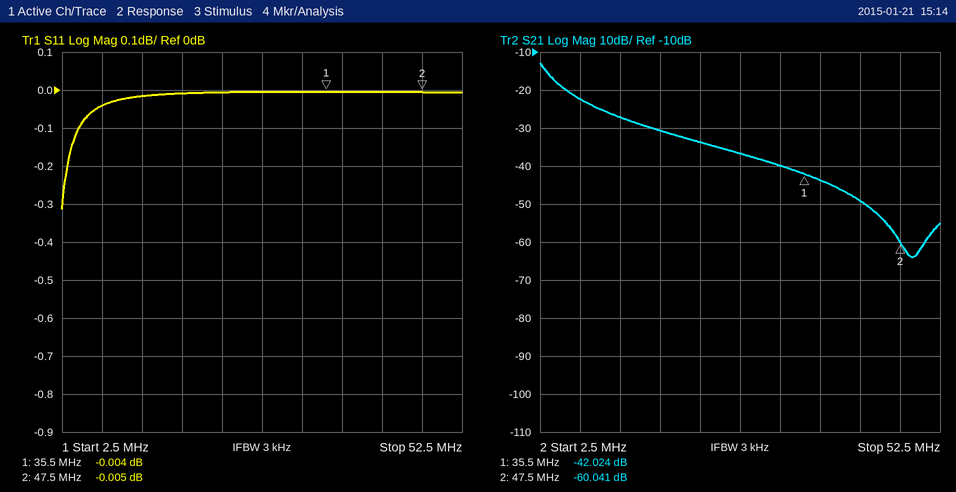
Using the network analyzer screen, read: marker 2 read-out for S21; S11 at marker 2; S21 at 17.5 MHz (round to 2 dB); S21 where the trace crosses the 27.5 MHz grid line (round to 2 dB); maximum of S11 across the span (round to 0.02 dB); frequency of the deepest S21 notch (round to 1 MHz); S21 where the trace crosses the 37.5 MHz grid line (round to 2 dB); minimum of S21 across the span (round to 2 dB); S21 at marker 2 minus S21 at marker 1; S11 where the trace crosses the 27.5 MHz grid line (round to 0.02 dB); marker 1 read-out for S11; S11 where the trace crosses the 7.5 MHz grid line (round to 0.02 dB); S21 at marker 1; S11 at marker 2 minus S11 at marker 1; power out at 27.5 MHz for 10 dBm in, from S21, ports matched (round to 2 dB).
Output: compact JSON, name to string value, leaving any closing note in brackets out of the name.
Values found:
{"marker 2 read-out for S21": "-60.041 dB", "S11 at marker 2": "-0.005 dB", "S21 at 17.5 MHz": "-30 dB", "S21 where the trace crosses the 27.5 MHz grid line": "-36 dB", "maximum of S11 across the span": "0.00 dB", "frequency of the deepest S21 notch": "49 MHz", "S21 where the trace crosses the 37.5 MHz grid line": "-44 dB", "minimum of S21 across the span": "-64 dB", "S21 at marker 2 minus S21 at marker 1": "-18.017 dB", "S11 where the trace crosses the 27.5 MHz grid line": "0.00 dB", "marker 1 read-out for S11": "-0.004 dB", "S11 where the trace crosses the 7.5 MHz grid line": "-0.04 dB", "S21 at marker 1": "-42.024 dB", "S11 at marker 2 minus S11 at marker 1": "-0.001 dB", "power out at 27.5 MHz for 10 dBm in, from S21, ports matched": "-26 dBm"}
